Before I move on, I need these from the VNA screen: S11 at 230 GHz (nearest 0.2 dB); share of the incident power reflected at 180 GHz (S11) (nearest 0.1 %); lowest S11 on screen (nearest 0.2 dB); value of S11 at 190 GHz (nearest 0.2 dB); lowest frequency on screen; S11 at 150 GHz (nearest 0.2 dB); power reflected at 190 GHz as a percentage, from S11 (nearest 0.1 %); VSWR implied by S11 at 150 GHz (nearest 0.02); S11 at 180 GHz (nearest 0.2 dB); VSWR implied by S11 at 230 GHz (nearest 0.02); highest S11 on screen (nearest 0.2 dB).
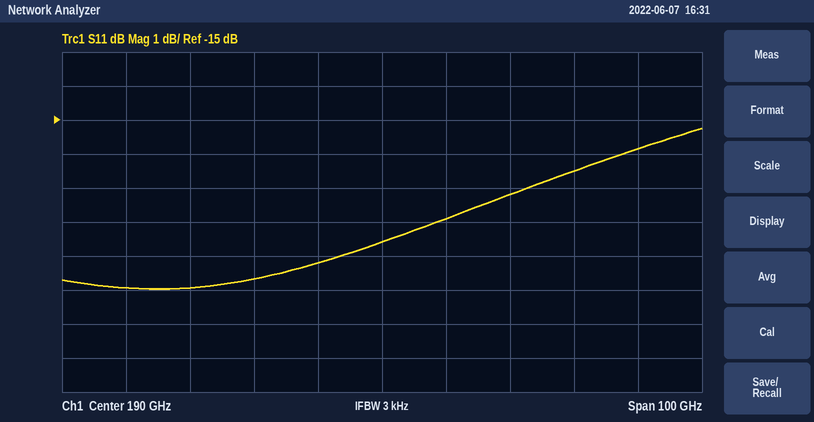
-15.8 dB
1.2 %
-20.0 dB
-18.6 dB
140 GHz
-20.0 dB
1.4 %
1.22
-19.2 dB
1.38
-15.2 dB
